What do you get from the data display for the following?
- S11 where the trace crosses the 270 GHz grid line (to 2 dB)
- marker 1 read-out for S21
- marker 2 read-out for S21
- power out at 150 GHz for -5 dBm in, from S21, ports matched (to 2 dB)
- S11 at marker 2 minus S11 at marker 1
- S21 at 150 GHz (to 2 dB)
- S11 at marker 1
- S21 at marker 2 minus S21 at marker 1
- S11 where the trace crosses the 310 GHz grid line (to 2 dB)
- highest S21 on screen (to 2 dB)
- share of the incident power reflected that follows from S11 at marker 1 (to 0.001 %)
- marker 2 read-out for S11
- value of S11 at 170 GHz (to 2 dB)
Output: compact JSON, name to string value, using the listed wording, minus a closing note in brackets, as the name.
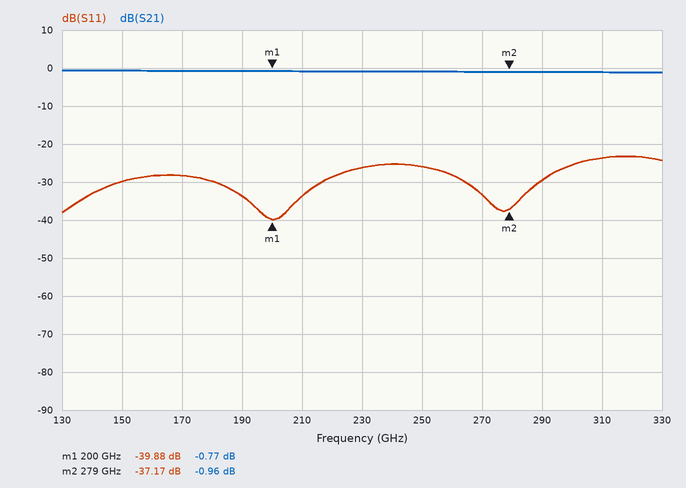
{"S11 where the trace crosses the 270 GHz grid line": "-34 dB", "marker 1 read-out for S21": "-0.77 dB", "marker 2 read-out for S21": "-0.96 dB", "power out at 150 GHz for -5 dBm in, from S21, ports matched": "-6 dBm", "S11 at marker 2 minus S11 at marker 1": "2.71 dB", "S21 at 150 GHz": "0 dB", "S11 at marker 1": "-39.88 dB", "S21 at marker 2 minus S21 at marker 1": "-0.19 dB", "S11 where the trace crosses the 310 GHz grid line": "-24 dB", "highest S21 on screen": "0 dB", "share of the incident power reflected that follows from S11 at marker 1": "0.010 %", "marker 2 read-out for S11": "-37.17 dB", "value of S11 at 170 GHz": "-28 dB"}
